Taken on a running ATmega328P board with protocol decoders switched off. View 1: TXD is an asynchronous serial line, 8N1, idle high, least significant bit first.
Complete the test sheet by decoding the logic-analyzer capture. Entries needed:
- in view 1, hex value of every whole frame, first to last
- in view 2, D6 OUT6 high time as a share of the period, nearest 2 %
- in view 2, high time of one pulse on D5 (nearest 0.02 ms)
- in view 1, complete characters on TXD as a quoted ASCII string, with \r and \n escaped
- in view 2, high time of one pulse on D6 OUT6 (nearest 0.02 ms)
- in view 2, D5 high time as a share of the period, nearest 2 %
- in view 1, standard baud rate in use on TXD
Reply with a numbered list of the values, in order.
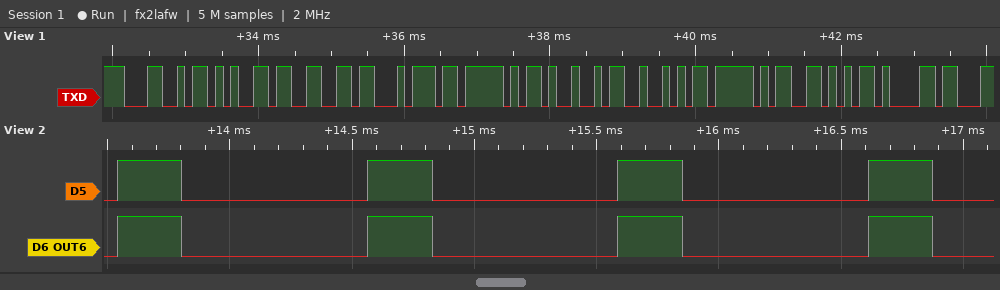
1. 0x4C 0x65 0x66 0x74 0x5F 0x49 0x52 0x5F 0x56 0x61
2. 26 %
3. 0.26 ms
4. "Left_IR_Va"
5. 0.26 ms
6. 26 %
7. 9600 baud
